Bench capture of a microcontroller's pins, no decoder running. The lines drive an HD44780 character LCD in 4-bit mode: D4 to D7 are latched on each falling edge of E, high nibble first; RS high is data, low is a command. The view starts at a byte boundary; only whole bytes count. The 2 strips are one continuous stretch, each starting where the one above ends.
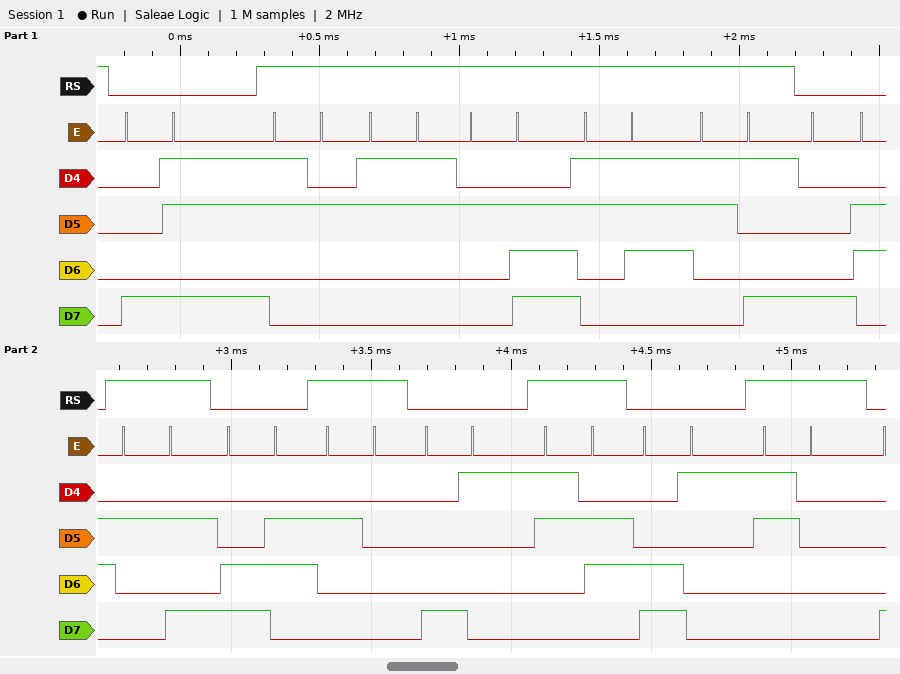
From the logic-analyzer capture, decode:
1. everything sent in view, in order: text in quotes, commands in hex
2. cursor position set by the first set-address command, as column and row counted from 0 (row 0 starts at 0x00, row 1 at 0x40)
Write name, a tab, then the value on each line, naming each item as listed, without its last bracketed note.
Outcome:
everything sent in view, in order: text in quotes, commands in hex	0x8B "23.79" 0x86 "*" 0xC6 " " 0x81 "6" 0xC1 "0"
cursor position set by the first set-address command, as column and row counted from 0	column 11, row 0
